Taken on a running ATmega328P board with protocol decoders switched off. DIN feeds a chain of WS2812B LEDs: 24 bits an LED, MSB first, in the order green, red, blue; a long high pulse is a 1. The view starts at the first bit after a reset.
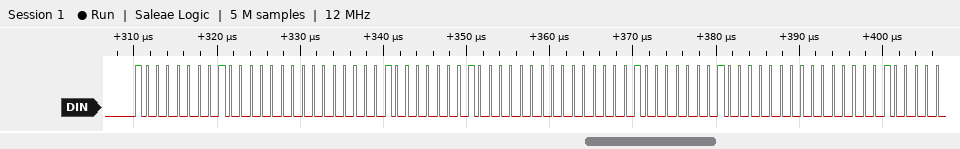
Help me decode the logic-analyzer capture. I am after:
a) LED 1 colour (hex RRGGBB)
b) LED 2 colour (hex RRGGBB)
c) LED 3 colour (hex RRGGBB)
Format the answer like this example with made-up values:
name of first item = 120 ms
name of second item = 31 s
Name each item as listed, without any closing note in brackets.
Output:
LED 1 colour = #808000
LED 2 colour = #808000
LED 3 colour = #808000
